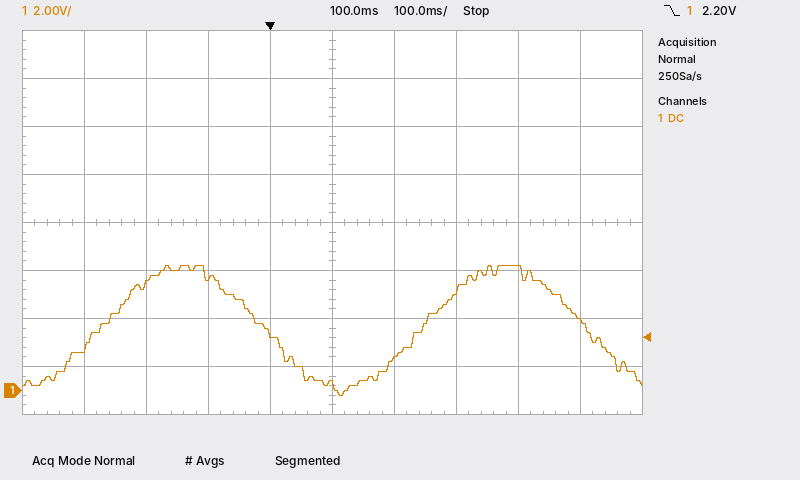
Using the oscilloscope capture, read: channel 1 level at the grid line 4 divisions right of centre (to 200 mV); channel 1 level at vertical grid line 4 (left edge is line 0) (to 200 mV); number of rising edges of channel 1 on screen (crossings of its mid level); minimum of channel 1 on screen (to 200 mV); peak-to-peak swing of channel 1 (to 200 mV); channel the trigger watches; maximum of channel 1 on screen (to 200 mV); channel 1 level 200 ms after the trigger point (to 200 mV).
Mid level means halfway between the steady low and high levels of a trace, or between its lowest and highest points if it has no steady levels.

3.0 V
2.4 V
2
-200 mV
5.4 V
channel 1
5.2 V
1.4 V
